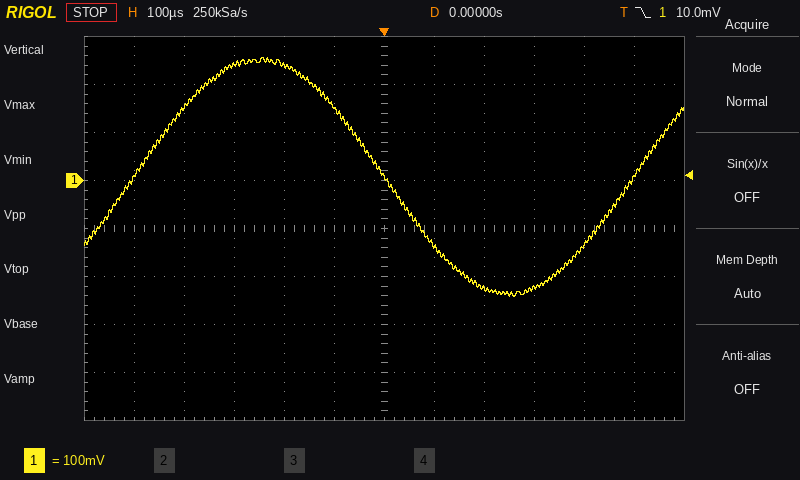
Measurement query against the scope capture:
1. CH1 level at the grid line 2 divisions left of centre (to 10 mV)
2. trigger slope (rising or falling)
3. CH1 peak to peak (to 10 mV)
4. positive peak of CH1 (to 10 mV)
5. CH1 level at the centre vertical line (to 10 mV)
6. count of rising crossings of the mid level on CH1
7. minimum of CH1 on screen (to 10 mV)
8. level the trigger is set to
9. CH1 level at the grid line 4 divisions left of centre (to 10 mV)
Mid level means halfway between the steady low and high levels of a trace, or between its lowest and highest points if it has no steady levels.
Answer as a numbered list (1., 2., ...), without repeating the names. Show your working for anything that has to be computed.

1. 240 mV
2. falling
3. 260 mV − (-240 mV) = 500 mV
4. 260 mV
5. 10 mV
6. 2
7. -240 mV
8. 10.0 mV
9. 150 mV
